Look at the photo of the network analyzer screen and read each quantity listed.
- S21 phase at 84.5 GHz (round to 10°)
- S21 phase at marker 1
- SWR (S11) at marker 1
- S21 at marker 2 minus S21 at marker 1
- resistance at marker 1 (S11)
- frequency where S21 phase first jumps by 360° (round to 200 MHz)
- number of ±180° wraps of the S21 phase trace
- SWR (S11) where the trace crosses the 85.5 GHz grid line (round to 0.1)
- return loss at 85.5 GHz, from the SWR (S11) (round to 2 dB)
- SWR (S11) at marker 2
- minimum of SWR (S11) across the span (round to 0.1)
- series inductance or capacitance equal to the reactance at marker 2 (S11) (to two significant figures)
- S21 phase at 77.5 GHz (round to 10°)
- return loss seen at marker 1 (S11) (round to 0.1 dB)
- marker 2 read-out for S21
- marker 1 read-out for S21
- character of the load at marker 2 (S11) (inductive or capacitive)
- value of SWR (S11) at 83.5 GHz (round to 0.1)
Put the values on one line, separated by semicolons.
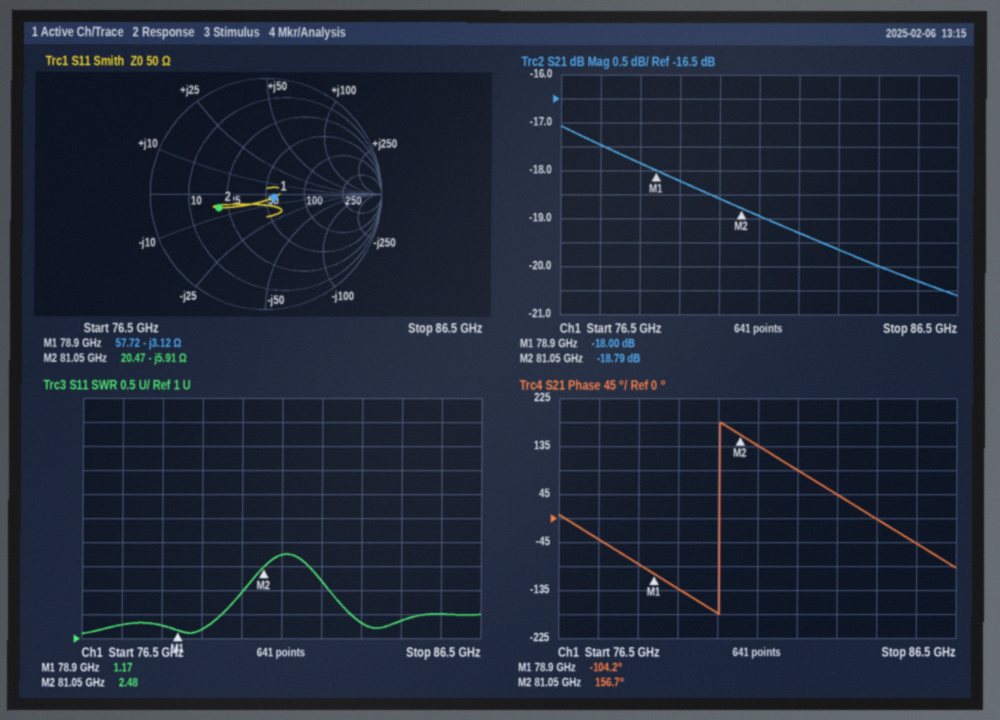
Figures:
0°; -104.2°; 1.17; -0.79 dB; 57.72 Ω; 80.6 GHz; 1; 1.5; 14 dB; 2.48; 1.1; 330 fF; -40°; 22.2 dB; -18.79 dB; -18.00 dB; capacitive; 1.3
